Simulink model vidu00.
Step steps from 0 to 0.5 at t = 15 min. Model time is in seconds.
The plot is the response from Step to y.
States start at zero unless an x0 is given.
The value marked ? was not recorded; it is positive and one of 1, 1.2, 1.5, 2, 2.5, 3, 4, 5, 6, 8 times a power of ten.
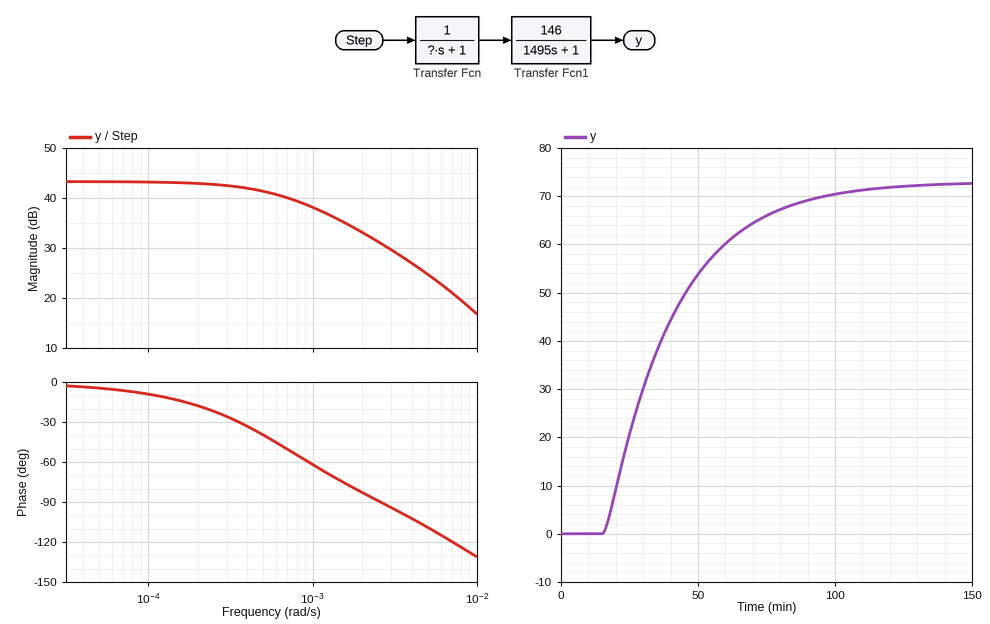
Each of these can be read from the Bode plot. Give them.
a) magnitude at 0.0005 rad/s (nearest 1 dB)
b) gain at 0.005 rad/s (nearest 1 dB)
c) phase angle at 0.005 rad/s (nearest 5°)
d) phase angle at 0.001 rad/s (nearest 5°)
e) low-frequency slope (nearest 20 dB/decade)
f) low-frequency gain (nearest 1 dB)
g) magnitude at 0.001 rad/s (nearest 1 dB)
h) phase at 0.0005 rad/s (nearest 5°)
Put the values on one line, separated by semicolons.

41 dB; 25 dB; -110°; -60°; 0 dB/decade; 43 dB; 38 dB; -40°
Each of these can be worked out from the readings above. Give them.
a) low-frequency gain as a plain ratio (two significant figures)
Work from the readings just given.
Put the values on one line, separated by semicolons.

140
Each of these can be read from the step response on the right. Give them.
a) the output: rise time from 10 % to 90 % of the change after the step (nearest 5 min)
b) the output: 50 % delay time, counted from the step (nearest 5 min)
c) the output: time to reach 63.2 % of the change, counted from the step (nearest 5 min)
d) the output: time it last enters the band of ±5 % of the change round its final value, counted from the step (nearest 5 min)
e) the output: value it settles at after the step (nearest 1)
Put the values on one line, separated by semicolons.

55 min; 20 min; 25 min; 75 min; 73
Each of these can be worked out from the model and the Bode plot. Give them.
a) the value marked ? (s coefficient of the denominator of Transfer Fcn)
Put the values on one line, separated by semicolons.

100
